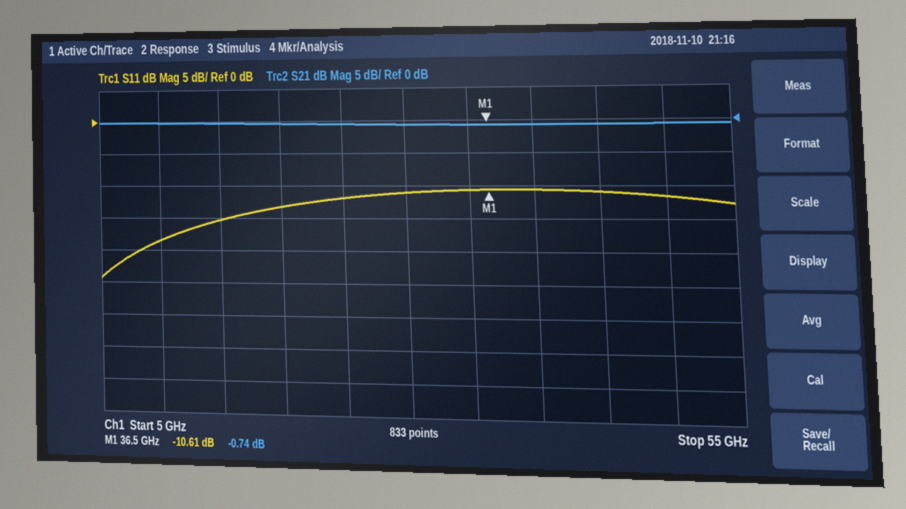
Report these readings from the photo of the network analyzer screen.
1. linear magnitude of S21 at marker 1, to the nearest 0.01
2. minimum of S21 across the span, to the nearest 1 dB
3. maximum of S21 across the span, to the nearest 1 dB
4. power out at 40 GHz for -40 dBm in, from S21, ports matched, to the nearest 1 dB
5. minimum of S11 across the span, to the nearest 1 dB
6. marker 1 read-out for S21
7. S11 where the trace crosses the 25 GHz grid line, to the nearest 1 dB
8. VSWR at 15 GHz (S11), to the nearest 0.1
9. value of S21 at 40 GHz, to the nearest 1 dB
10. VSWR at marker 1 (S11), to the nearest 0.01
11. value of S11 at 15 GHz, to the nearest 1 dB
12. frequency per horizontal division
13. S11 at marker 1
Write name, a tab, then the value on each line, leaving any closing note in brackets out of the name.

linear magnitude of S21 at marker 1, to the nearest 0.01	0.92
minimum of S21 across the span, to the nearest 1 dB	-1 dB
maximum of S21 across the span, to the nearest 1 dB	0 dB
power out at 40 GHz for -40 dBm in, from S21, ports matched, to the nearest 1 dB	-41 dBm
minimum of S11 across the span, to the nearest 1 dB	-24 dB
marker 1 read-out for S21	-0.74 dB
S11 where the trace crosses the 25 GHz grid line, to the nearest 1 dB	-12 dB
VSWR at 15 GHz (S11), to the nearest 0.1	1.4
value of S21 at 40 GHz, to the nearest 1 dB	-1 dB
VSWR at marker 1 (S11), to the nearest 0.01	1.84
value of S11 at 15 GHz, to the nearest 1 dB	-15 dB
frequency per horizontal division	5 GHz
S11 at marker 1	-10.61 dB
